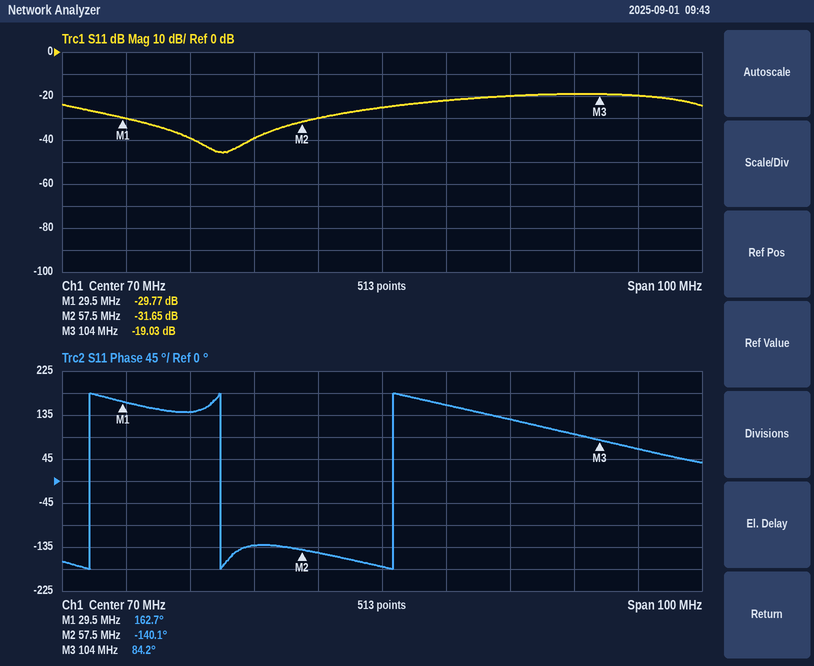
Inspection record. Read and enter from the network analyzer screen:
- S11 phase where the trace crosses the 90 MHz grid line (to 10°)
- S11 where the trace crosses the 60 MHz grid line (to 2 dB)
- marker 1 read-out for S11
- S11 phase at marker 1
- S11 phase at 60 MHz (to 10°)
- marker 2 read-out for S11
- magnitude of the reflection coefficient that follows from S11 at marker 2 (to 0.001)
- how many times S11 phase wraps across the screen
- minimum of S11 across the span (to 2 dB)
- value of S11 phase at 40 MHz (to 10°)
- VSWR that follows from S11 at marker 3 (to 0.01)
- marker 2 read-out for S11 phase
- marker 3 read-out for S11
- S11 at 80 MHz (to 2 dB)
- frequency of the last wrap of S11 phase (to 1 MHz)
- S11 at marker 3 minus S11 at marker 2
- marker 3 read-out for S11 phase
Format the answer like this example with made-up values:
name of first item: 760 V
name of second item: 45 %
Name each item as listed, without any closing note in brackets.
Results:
S11 phase where the trace crosses the 90 MHz grid line: 130°
S11 where the trace crosses the 60 MHz grid line: -30 dB
marker 1 read-out for S11: -29.77 dB
S11 phase at marker 1: 162.7°
S11 phase at 60 MHz: -150°
marker 2 read-out for S11: -31.65 dB
magnitude of the reflection coefficient that follows from S11 at marker 2: 0.026
how many times S11 phase wraps across the screen: 3
minimum of S11 across the span: -46 dB
value of S11 phase at 40 MHz: 140°
VSWR that follows from S11 at marker 3: 1.25
marker 2 read-out for S11 phase: -140.1°
marker 3 read-out for S11: -19.03 dB
S11 at 80 MHz: -22 dB
frequency of the last wrap of S11 phase: 72 MHz
S11 at marker 3 minus S11 at marker 2: 12.62 dB
marker 3 read-out for S11 phase: 84.2°
